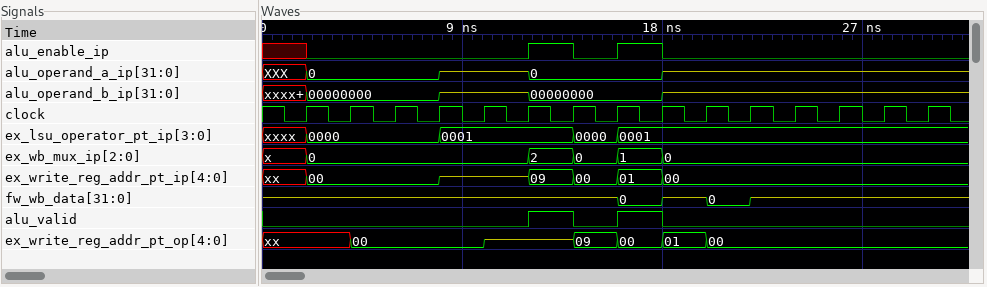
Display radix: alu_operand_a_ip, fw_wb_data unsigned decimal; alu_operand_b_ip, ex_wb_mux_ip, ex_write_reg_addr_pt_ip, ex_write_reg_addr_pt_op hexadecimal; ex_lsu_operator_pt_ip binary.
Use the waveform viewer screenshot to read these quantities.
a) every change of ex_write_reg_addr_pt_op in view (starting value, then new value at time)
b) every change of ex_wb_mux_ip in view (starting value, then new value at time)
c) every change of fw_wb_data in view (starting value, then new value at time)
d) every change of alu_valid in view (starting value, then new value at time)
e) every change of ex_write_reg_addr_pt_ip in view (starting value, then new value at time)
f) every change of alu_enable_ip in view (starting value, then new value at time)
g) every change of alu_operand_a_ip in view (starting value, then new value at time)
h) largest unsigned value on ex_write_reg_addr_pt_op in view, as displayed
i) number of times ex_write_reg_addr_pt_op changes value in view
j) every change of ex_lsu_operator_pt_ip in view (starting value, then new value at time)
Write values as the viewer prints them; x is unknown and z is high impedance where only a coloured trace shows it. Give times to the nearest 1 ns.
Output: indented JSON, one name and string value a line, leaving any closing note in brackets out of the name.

{
  "every change of ex_write_reg_addr_pt_op in view": "xx, 00 at 4 ns, z at 10 ns, 09 at 14 ns, 00 at 16 ns, 01 at 18 ns, 00 at 20 ns",
  "every change of ex_wb_mux_ip in view": "x, 0 at 2 ns, 2 at 12 ns, 0 at 14 ns, 1 at 16 ns, 0 at 18 ns",
  "every change of fw_wb_data in view": "z, 0 at 16 ns, z at 18 ns, 0 at 20 ns, z at 22 ns",
  "every change of alu_valid in view": "0, 1 at 12 ns, 0 at 14 ns, 1 at 16 ns, 0 at 18 ns",
  "every change of ex_write_reg_addr_pt_ip in view": "xx, 00 at 2 ns, z at 8 ns, 09 at 12 ns, 00 at 14 ns, 01 at 16 ns, 00 at 18 ns",
  "every change of alu_enable_ip in view": "x, 0 at 2 ns, 1 at 12 ns, 0 at 14 ns, 1 at 16 ns, 0 at 18 ns",
  "every change of alu_operand_a_ip in view": "XXX, 0 at 2 ns, z at 8 ns, 0 at 12 ns, z at 18 ns",
  "largest unsigned value on ex_write_reg_addr_pt_op in view, as displayed": "09",
  "number of times ex_write_reg_addr_pt_op changes value in view": "6",
  "every change of ex_lsu_operator_pt_ip in view": "xxxx, 0000 at 2 ns, 0001 at 8 ns, 0000 at 14 ns, 0001 at 16 ns"
}
